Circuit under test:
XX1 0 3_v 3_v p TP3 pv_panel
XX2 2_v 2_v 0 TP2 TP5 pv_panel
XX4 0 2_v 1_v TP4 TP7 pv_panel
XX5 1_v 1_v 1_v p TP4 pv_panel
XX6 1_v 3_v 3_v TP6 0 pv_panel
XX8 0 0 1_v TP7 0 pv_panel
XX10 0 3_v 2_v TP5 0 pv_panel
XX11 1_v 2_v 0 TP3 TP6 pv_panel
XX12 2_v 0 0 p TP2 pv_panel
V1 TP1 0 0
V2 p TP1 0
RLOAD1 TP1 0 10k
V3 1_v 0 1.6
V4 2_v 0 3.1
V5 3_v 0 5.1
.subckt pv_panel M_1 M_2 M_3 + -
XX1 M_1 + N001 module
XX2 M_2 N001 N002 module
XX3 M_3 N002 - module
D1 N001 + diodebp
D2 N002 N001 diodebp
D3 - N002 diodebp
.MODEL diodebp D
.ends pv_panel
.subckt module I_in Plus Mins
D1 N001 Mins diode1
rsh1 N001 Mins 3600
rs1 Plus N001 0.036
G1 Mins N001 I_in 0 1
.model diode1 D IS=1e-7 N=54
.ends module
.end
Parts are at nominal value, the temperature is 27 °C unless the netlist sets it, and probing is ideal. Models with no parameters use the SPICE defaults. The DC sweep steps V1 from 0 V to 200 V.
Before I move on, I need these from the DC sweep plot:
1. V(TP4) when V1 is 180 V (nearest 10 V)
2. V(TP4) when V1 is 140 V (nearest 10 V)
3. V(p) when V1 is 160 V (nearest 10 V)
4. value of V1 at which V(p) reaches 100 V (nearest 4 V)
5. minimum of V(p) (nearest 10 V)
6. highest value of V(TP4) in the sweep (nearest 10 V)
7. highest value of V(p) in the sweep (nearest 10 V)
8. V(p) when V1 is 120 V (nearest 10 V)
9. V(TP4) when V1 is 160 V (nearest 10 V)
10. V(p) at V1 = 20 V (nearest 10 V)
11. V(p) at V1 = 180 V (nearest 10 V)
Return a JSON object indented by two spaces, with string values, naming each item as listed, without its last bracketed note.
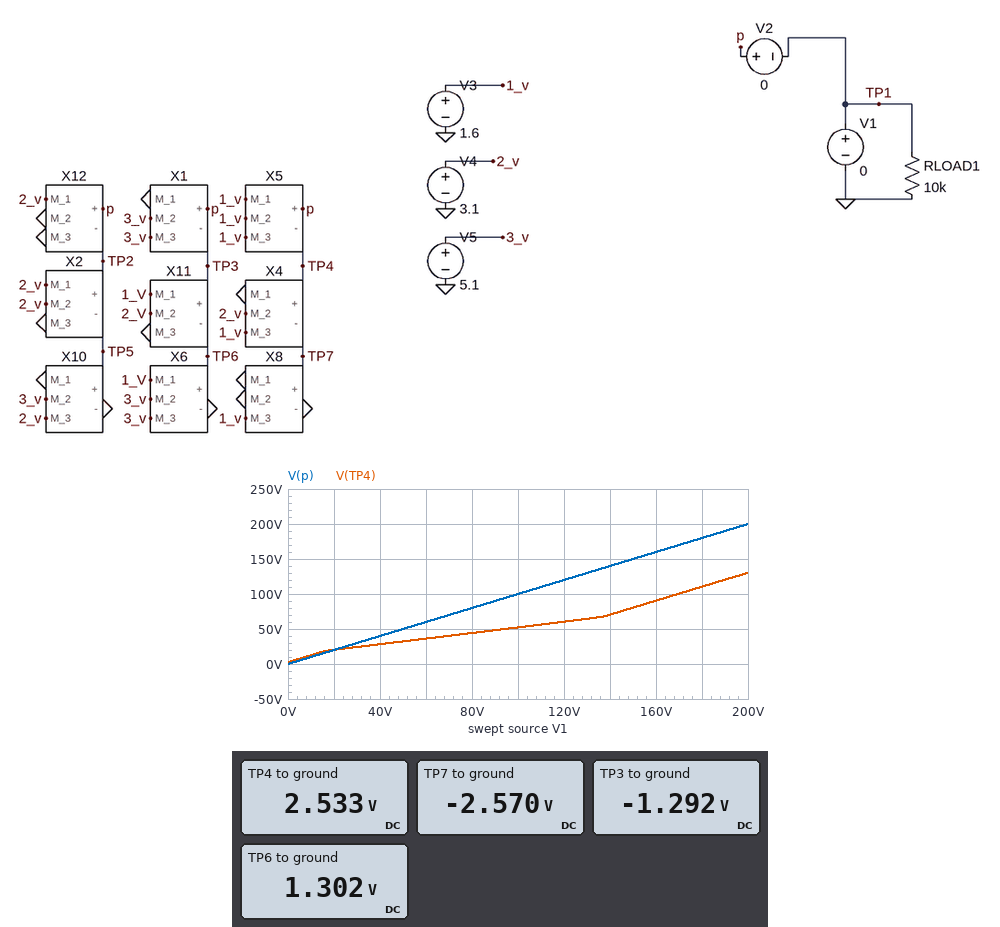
{
  "V(TP4) when V1 is 180 V": "110 V",
  "V(TP4) when V1 is 140 V": "70 V",
  "V(p) when V1 is 160 V": "160 V",
  "value of V1 at which V(p) reaches 100 V": "100 V",
  "minimum of V(p)": "0 V",
  "highest value of V(TP4) in the sweep": "130 V",
  "highest value of V(p) in the sweep": "200 V",
  "V(p) when V1 is 120 V": "120 V",
  "V(TP4) when V1 is 160 V": "90 V",
  "V(p) at V1 = 20 V": "20 V",
  "V(p) at V1 = 180 V": "180 V"
}
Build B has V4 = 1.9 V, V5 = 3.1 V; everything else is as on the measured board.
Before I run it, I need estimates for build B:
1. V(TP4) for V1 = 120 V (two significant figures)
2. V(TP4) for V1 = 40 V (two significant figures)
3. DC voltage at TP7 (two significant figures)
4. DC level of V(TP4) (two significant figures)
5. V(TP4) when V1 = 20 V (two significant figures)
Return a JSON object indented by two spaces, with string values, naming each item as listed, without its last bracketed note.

{
  "V(TP4) for V1 = 120 V": "59 V",
  "V(TP4) for V1 = 40 V": "27 V",
  "DC voltage at TP7": "-2.5 V",
  "DC level of V(TP4)": "2.4 V",
  "V(TP4) when V1 = 20 V": "19 V"
}
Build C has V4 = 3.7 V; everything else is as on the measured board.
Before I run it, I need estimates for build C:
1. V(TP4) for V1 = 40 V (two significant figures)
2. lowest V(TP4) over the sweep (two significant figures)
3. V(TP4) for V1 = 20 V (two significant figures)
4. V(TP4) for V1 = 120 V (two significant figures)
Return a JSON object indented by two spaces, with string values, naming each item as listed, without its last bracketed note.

{
  "V(TP4) for V1 = 40 V": "29 V",
  "lowest V(TP4) over the sweep": "2.6 V",
  "V(TP4) for V1 = 20 V": "21 V",
  "V(TP4) for V1 = 120 V": "61 V"
}
